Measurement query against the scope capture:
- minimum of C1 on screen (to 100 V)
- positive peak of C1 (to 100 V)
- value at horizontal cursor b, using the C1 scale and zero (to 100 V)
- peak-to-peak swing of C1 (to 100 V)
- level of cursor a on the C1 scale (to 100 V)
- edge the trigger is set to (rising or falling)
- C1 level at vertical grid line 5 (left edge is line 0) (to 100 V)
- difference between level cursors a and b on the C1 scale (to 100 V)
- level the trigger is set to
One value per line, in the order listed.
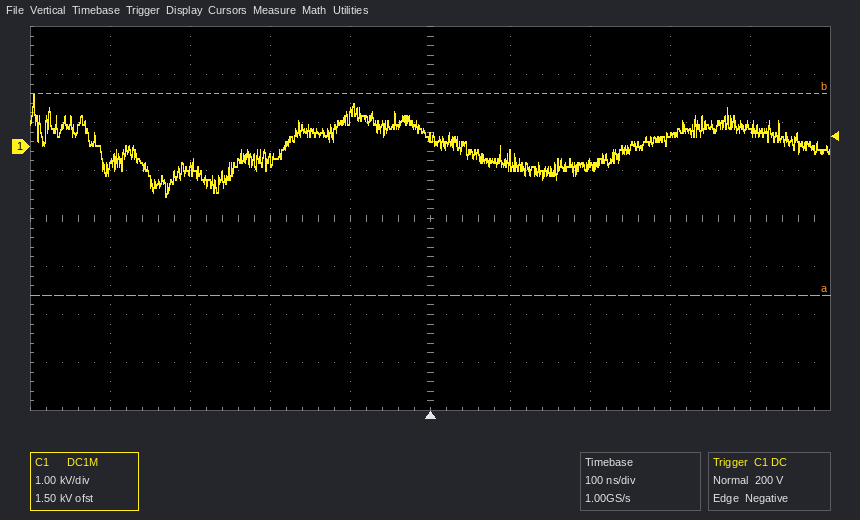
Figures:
-1.0 kV
1.1 kV
1.1 kV
2.1 kV
-3.1 kV
falling
200 V
4.2 kV
200 V
